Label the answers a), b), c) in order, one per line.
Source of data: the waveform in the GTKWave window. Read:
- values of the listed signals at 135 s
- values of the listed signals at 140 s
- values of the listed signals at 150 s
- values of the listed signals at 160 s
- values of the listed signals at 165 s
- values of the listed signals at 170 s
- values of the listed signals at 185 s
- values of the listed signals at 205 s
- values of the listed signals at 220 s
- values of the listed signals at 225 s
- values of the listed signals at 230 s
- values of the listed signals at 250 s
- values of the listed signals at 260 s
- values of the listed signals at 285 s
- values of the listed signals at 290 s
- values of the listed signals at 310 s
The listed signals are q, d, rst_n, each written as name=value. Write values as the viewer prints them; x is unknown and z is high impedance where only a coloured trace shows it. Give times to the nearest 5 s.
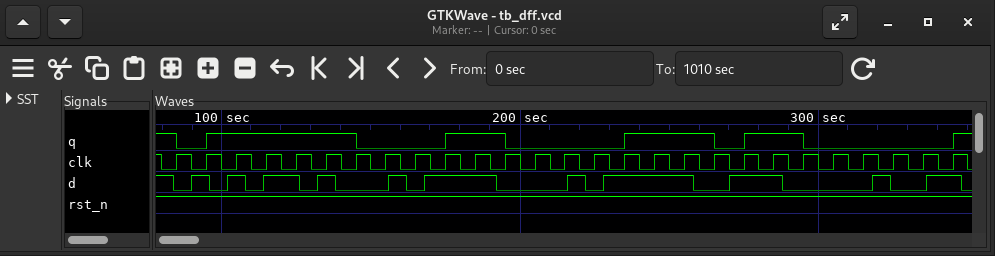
a) q=1, d=1, rst_n=1
b) q=1, d=0, rst_n=1
c) q=0, d=0, rst_n=1
d) q=0, d=1, rst_n=1
e) q=0, d=0, rst_n=1
f) q=0, d=1, rst_n=1
g) q=1, d=1, rst_n=1
h) q=0, d=0, rst_n=1
i) q=0, d=1, rst_n=1
j) q=0, d=0, rst_n=1
k) q=0, d=1, rst_n=1
l) q=1, d=1, rst_n=1
m) q=1, d=0, rst_n=1
n) q=1, d=1, rst_n=1
o) q=1, d=0, rst_n=1
p) q=0, d=0, rst_n=1
